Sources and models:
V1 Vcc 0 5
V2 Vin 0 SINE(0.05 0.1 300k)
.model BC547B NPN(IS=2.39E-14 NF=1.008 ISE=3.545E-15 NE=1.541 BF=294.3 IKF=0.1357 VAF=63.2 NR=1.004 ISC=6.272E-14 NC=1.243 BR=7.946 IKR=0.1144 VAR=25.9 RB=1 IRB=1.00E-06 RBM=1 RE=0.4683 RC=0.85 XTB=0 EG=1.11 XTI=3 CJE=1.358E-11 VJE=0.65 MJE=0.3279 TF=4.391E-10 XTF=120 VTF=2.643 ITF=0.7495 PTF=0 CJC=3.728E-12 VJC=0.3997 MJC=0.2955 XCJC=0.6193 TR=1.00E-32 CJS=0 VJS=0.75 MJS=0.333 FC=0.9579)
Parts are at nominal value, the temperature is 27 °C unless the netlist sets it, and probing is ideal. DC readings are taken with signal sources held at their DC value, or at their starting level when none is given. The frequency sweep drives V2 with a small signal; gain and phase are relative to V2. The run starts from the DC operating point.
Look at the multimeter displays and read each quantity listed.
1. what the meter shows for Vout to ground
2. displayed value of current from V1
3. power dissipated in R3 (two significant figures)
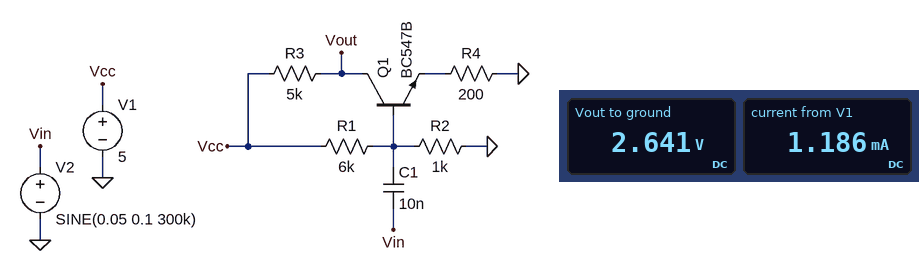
2.641 V
1.186 mA
1.1 mW
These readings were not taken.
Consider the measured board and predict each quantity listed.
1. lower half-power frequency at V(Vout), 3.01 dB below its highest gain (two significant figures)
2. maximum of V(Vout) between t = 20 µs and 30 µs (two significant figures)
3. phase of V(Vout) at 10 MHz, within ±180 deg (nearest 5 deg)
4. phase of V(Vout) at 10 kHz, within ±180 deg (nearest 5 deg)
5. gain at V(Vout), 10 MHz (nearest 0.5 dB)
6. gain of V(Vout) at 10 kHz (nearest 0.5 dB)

19 kHz
4.3 V
135 deg
-120 deg
24.0 dB
19.0 dB
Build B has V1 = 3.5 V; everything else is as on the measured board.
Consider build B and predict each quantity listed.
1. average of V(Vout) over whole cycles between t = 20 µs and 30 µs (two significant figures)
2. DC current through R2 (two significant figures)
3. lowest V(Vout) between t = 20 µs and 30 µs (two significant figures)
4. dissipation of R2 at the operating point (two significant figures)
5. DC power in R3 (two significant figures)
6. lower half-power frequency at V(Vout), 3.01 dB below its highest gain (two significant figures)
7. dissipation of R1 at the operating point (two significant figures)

3.4 V
500 µA
3.0 V
250 µW
130 nW
31 kHz
1.5 mW
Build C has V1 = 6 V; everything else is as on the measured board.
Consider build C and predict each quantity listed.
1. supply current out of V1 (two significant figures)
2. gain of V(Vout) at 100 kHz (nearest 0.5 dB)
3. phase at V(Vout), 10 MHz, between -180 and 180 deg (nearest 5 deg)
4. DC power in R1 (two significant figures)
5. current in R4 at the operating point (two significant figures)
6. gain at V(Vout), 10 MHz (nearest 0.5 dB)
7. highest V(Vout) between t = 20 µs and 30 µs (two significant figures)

1.9 mA
26.5 dB
120 deg
4.4 mW
1.1 mA
22.0 dB
3.4 V
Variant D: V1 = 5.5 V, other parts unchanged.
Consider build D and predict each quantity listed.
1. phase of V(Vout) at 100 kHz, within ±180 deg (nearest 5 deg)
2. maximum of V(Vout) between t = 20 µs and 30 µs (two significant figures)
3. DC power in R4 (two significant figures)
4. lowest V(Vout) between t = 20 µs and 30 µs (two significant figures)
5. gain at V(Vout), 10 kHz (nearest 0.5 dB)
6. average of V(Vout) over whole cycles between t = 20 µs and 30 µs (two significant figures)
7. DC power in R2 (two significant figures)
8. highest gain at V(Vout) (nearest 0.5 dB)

-170 deg
3.8 V
120 µW
260 mV
20.0 dB
1.9 V
610 µW
26.5 dB
